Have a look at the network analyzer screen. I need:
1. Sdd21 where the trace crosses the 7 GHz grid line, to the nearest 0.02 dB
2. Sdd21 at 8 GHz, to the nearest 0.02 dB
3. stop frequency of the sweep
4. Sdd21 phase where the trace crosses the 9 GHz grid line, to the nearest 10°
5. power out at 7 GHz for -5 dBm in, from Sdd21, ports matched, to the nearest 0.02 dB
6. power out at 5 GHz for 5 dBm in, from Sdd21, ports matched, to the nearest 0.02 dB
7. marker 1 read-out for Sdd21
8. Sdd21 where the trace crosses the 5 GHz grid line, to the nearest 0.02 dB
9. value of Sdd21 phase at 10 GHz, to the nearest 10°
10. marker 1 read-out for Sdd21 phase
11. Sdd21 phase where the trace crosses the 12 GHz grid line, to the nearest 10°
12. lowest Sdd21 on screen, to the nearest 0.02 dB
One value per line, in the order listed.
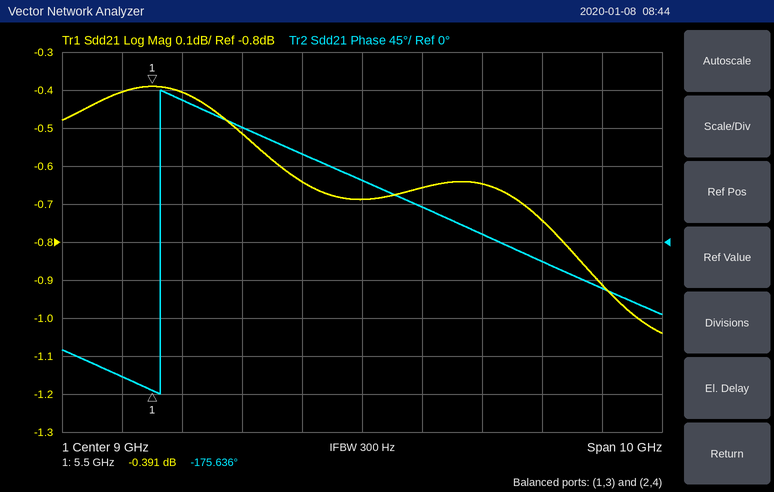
-0.52 dB
-0.64 dB
14 GHz
70°
-5.52 dBm
4.60 dBm
-0.391 dB
-0.40 dB
40°
-175.636°
-20°
-1.04 dB
